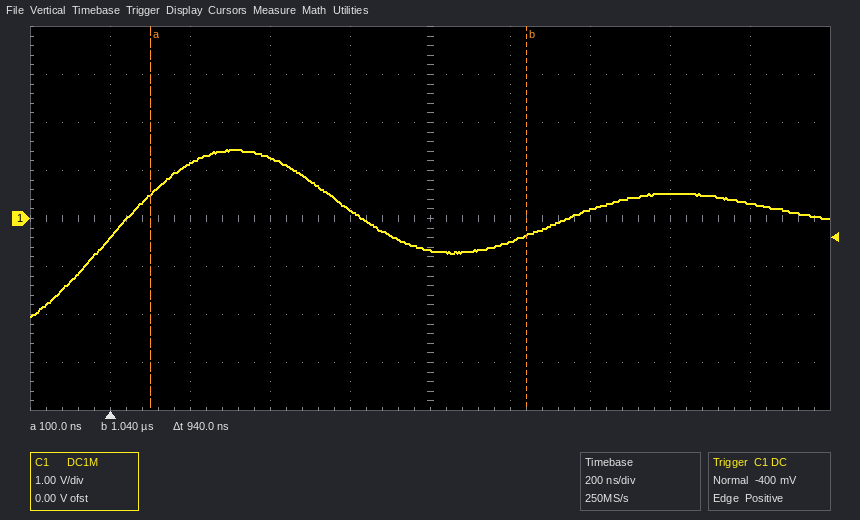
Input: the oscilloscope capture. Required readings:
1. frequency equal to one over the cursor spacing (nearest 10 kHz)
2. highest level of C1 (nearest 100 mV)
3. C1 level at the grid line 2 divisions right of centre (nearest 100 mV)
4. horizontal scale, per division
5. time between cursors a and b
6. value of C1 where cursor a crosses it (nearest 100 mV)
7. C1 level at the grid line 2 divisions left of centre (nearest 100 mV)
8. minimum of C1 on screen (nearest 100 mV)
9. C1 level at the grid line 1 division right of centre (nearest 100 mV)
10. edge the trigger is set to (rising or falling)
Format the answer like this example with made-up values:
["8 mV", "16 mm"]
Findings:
["1.06 MHz", "1.4 V", "200 mV", "200 ns", "940 ns", "500 mV", "1.3 V", "-2.0 V", "-500 mV", "rising"]
